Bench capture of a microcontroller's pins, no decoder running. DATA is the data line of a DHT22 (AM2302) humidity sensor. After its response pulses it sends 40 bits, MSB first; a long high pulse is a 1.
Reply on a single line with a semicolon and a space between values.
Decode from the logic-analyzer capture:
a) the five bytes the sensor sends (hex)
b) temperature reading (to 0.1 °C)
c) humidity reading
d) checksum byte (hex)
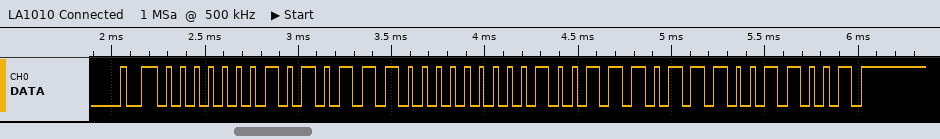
01 5C 01 3B 99; 31.5 °C; 34.8 %; 0x99
